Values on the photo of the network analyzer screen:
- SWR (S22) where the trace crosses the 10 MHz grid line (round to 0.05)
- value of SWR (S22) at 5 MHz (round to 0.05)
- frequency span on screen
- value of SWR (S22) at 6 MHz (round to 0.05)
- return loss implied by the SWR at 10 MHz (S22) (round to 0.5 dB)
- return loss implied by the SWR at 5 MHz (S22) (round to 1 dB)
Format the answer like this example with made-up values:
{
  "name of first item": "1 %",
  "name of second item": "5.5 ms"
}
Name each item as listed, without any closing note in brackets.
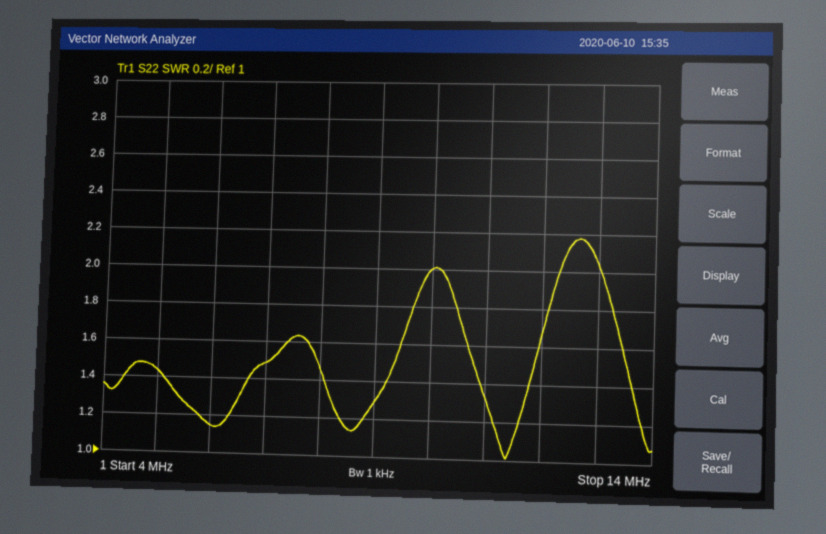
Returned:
{
  "SWR (S22) where the trace crosses the 10 MHz grid line": "2.00",
  "value of SWR (S22) at 5 MHz": "1.45",
  "frequency span on screen": "10 MHz",
  "value of SWR (S22) at 6 MHz": "1.15",
  "return loss implied by the SWR at 10 MHz (S22)": "9.5 dB",
  "return loss implied by the SWR at 5 MHz (S22)": "15 dB"
}
